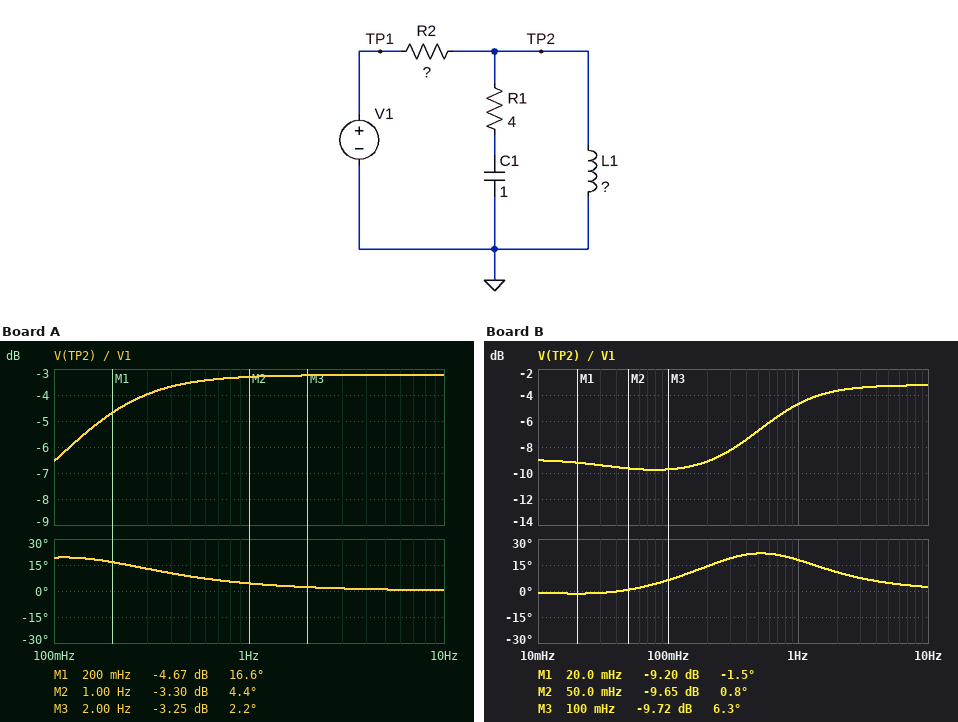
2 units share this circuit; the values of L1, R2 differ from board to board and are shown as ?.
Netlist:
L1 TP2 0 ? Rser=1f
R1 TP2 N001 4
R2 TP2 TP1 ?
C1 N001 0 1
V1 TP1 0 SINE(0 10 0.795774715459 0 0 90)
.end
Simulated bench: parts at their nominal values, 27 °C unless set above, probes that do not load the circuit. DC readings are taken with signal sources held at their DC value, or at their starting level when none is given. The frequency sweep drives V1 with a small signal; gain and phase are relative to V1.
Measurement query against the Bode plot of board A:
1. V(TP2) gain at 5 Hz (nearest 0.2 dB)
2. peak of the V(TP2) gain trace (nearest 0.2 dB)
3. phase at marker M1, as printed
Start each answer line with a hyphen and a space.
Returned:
- -3.2 dB
- -3.2 dB
- 16.6 deg
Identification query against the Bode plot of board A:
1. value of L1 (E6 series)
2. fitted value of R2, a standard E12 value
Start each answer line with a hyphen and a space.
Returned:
- 2.2 H
- 1.8 Ω
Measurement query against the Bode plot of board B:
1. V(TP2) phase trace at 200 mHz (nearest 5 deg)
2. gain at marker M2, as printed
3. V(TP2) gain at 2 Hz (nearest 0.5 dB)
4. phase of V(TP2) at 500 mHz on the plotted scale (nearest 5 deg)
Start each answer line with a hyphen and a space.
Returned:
- 15 deg
- -9.65 dB
- -3.5 dB
- 20 deg
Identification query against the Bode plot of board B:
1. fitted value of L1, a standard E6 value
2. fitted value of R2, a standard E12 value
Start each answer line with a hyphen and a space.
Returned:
- 470 mH
- 1.8 Ω
